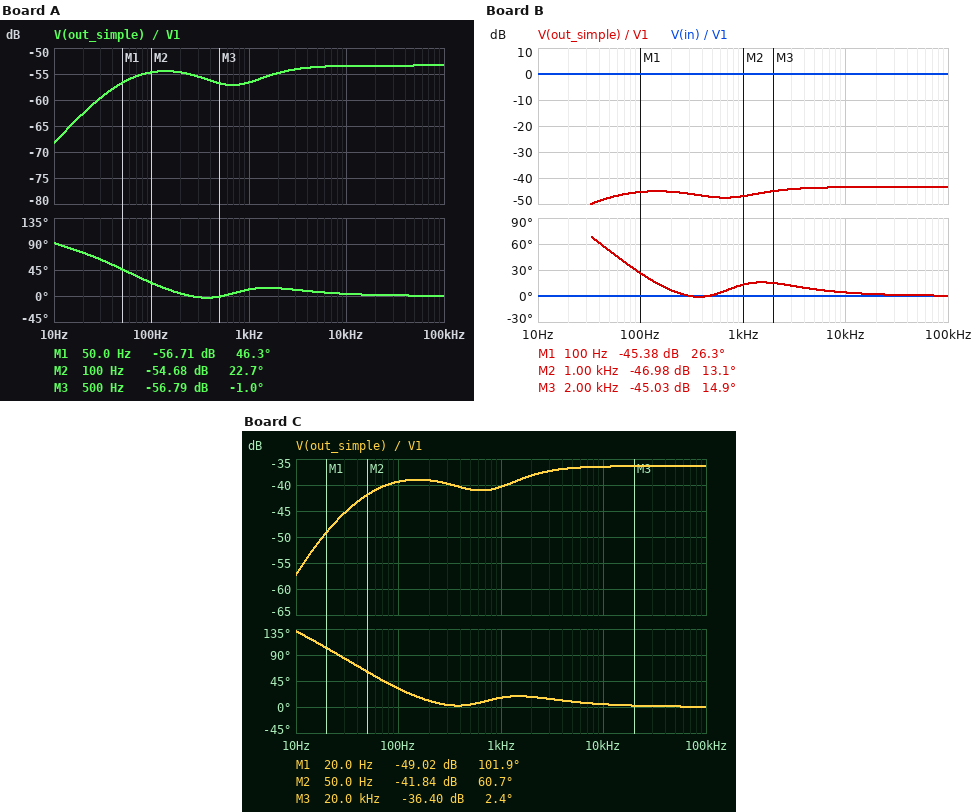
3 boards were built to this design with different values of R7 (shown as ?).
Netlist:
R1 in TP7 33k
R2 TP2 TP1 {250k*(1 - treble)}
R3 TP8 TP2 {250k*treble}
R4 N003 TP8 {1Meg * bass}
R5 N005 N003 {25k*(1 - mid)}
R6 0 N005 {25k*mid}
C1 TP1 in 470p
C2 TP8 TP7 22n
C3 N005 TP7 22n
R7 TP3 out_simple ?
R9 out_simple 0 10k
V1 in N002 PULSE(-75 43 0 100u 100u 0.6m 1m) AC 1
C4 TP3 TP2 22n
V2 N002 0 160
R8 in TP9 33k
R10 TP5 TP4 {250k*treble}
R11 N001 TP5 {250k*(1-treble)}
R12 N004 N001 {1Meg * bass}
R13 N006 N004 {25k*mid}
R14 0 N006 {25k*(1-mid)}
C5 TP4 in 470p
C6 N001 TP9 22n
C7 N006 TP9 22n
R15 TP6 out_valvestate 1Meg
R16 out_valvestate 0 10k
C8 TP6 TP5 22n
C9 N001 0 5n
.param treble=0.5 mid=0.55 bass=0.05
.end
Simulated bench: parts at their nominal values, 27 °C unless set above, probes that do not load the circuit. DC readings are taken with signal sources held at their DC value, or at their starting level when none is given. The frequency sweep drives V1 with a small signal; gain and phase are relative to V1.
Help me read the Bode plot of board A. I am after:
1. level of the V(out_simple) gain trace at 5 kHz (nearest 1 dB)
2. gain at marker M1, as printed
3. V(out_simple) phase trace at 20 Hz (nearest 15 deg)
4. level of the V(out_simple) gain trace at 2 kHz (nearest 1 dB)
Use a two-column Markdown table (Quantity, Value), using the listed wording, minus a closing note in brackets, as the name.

| Quantity | Value |
|---|---|
| level of the V(out_simple) gain trace at 5 kHz | -54 dB |
| gain at marker M1, as printed | -56.71 dB |
| V(out_simple) phase trace at 20 Hz | 75 deg |
| level of the V(out_simple) gain trace at 2 kHz | -55 dB |
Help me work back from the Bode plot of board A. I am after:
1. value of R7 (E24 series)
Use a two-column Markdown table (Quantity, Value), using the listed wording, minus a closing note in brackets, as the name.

| Quantity | Value |
|---|---|
| value of R7 | 3 MΩ |
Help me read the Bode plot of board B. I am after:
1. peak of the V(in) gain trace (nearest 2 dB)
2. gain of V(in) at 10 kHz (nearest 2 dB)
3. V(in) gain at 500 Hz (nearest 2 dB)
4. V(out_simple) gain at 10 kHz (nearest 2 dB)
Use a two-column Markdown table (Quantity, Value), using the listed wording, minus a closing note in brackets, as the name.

| Quantity | Value |
|---|---|
| peak of the V(in) gain trace | 0 dB |
| gain of V(in) at 10 kHz | 0 dB |
| V(in) gain at 500 Hz | 0 dB |
| V(out_simple) gain at 10 kHz | -44 dB |
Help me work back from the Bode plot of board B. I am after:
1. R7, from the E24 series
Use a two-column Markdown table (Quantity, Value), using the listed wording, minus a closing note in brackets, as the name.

| Quantity | Value |
|---|---|
| R7, from the E24 series | 910 kΩ |
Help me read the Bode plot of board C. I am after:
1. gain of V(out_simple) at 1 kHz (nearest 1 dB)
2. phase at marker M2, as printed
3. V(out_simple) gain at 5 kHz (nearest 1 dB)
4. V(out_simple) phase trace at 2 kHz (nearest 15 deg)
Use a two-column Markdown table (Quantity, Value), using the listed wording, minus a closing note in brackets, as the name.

| Quantity | Value |
|---|---|
| gain of V(out_simple) at 1 kHz | -40 dB |
| phase at marker M2, as printed | 60.7 deg |
| V(out_simple) gain at 5 kHz | -37 dB |
| V(out_simple) phase trace at 2 kHz | 15 deg |
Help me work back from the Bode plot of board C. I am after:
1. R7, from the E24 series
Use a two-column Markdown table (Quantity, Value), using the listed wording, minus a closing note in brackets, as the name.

| Quantity | Value |
|---|---|
| R7, from the E24 series | 360 kΩ |
